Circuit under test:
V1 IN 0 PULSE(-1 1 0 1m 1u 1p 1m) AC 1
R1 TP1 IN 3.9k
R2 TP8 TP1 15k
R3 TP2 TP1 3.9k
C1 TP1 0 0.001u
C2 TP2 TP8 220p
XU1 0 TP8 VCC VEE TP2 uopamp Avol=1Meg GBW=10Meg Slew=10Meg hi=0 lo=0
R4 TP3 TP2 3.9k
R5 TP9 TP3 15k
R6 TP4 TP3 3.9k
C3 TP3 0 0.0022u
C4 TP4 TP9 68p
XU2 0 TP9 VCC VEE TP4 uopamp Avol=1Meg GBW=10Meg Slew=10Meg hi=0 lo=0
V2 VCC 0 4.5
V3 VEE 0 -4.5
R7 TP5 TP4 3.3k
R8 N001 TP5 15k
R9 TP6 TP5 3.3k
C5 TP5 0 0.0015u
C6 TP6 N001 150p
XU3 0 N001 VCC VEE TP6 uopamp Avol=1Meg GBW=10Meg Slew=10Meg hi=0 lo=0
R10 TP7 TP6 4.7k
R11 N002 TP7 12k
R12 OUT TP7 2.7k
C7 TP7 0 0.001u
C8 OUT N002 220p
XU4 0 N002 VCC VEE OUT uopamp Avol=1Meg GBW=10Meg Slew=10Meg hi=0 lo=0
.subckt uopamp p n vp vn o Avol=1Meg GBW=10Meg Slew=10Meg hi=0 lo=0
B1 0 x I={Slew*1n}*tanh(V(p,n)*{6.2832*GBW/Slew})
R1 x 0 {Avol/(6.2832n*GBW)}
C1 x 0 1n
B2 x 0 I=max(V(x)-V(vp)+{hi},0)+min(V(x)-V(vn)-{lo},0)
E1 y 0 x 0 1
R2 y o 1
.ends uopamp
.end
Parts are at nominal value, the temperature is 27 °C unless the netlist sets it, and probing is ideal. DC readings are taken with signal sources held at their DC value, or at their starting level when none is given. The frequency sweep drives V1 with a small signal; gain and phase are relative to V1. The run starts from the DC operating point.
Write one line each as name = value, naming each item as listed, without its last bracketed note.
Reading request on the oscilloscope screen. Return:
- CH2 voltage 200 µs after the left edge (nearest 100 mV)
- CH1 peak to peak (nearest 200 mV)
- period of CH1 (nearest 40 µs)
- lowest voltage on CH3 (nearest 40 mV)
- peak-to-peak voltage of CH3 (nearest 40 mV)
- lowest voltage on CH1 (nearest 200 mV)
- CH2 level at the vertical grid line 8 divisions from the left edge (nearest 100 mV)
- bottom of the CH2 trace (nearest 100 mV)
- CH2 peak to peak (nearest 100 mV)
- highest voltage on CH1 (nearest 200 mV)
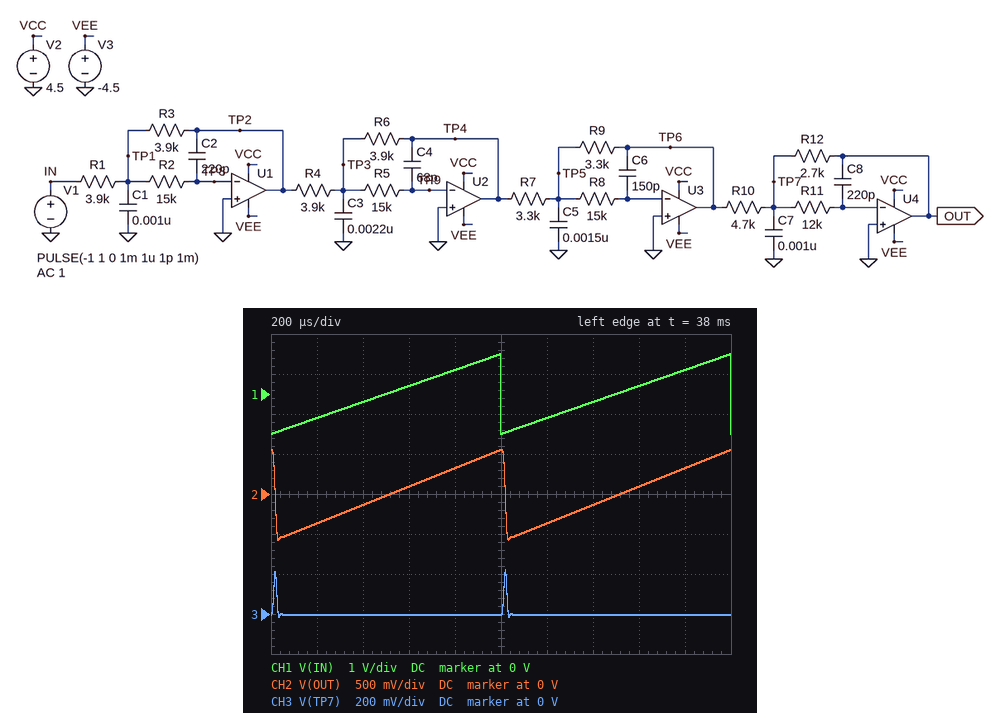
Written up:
CH2 voltage 200 µs after the left edge = -400 mV
CH1 peak to peak = 2.0 V
period of CH1 = 1.00 ms
lowest voltage on CH3 = 0 V
peak-to-peak voltage of CH3 = 240 mV
lowest voltage on CH1 = -1.0 V
CH2 level at the vertical grid line 8 divisions from the left edge = 100 mV
bottom of the CH2 trace = -600 mV
CH2 peak to peak = 1.1 V
highest voltage on CH1 = 1.0 V
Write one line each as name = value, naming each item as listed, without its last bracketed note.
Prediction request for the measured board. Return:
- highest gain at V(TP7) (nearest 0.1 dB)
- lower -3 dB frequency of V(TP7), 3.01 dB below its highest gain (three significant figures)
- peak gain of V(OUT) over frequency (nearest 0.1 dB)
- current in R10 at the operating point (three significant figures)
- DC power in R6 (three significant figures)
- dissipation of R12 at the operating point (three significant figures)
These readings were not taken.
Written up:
highest gain at V(TP7) = -14.9 dB
lower -3 dB frequency of V(TP7), 3.01 dB below its highest gain = 15.0 kHz
peak gain of V(OUT) over frequency = -4.8 dB
current in R10 at the operating point = 213 µA
DC power in R6 = 256 µW
dissipation of R12 at the operating point = 122 µW
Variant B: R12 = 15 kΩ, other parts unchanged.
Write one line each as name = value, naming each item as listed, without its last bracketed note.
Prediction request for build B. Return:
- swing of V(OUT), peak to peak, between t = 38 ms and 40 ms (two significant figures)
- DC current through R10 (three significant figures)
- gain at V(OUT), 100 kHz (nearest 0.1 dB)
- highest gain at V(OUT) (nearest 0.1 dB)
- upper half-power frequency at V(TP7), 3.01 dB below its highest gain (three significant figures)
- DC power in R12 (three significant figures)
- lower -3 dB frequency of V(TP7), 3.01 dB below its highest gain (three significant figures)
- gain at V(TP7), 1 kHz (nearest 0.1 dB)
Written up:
swing of V(OUT), peak to peak, between t = 38 ms and 40 ms = 5.9 V
DC current through R10 = 213 µA
gain at V(OUT), 100 kHz = -53.2 dB
highest gain at V(OUT) = 10.1 dB
upper half-power frequency at V(TP7), 3.01 dB below its highest gain = 36.1 kHz
DC power in R12 = 679 µW
lower -3 dB frequency of V(TP7), 3.01 dB below its highest gain = 7.79 kHz
gain at V(TP7), 1 kHz = -25.5 dB
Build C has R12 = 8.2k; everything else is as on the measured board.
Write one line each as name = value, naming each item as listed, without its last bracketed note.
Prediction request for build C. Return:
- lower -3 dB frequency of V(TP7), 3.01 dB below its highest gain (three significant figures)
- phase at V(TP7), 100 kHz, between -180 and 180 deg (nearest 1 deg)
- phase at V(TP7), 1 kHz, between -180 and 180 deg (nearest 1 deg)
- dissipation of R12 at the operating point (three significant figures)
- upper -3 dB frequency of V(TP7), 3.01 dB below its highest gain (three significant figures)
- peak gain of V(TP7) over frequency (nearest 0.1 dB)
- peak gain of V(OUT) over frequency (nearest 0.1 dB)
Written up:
lower -3 dB frequency of V(TP7), 3.01 dB below its highest gain = 10.8 kHz
phase at V(TP7), 100 kHz, between -180 and 180 deg = 67 deg
phase at V(TP7), 1 kHz, between -180 and 180 deg = -99 deg
dissipation of R12 at the operating point = 371 µW
upper -3 dB frequency of V(TP7), 3.01 dB below its highest gain = 40.7 kHz
peak gain of V(TP7) over frequency = -8.2 dB
peak gain of V(OUT) over frequency = 4.8 dB
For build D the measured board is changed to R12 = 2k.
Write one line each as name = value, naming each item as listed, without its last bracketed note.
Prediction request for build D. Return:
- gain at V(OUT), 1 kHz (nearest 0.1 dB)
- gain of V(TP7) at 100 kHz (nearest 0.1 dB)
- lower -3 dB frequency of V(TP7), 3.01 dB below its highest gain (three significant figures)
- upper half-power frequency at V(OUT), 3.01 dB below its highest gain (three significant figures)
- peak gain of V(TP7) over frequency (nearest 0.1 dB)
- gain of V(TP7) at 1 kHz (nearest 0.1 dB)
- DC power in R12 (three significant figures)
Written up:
gain at V(OUT), 1 kHz = -7.4 dB
gain of V(TP7) at 100 kHz = -50.6 dB
lower -3 dB frequency of V(TP7), 3.01 dB below its highest gain = 15.5 kHz
upper half-power frequency at V(OUT), 3.01 dB below its highest gain = 26.4 kHz
peak gain of V(TP7) over frequency = -17.2 dB
gain of V(TP7) at 1 kHz = -43.0 dB
DC power in R12 = 90.5 µW
